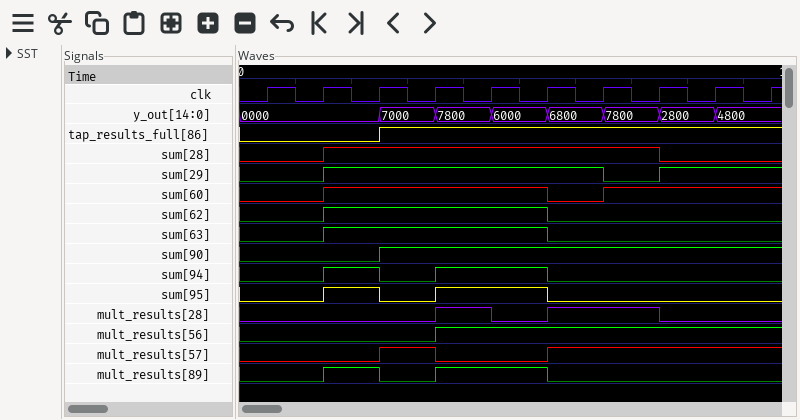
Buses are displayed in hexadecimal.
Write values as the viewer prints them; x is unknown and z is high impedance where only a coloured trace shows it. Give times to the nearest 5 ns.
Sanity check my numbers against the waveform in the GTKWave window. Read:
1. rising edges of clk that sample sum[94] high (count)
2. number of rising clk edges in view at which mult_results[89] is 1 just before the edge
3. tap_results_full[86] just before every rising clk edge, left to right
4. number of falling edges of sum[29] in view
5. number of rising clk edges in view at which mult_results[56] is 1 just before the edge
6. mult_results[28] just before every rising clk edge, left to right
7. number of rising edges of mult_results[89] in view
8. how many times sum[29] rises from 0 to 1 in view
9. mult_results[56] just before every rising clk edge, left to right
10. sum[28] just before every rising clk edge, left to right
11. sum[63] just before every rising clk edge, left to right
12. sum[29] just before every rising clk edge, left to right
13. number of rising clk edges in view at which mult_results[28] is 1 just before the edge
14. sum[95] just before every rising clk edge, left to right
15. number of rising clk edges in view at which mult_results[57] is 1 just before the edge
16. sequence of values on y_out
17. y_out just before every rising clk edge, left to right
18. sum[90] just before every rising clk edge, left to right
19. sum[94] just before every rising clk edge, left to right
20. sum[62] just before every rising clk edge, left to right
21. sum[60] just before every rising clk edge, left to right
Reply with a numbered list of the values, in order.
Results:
1. 3
2. 3
3. 0 0 0 1 1 1 1 1 1 1
4. 1
5. 6
6. 0 0 0 0 1 0 1 1 0 0
7. 2
8. 2
9. 0 0 0 0 1 1 1 1 1 1
10. 0 0 1 1 1 1 1 1 0 0
11. 0 0 1 1 1 1 0 0 0 0
12. 0 0 1 1 1 1 1 0 1 1
13. 3
14. 0 0 1 0 1 1 0 0 0 0
15. 5
16. 0000, 7000, 7800, 6000, 6800, 7800, 2800, 4800
17. 0000, 0000, 0000, 7000, 7800, 6000, 6800, 7800, 2800, 4800
18. 0 0 0 1 1 1 1 1 1 1
19. 0 0 1 0 1 1 0 0 0 0
20. 0 0 1 1 1 1 0 0 0 0
21. 0 0 1 1 1 1 0 1 1 1
